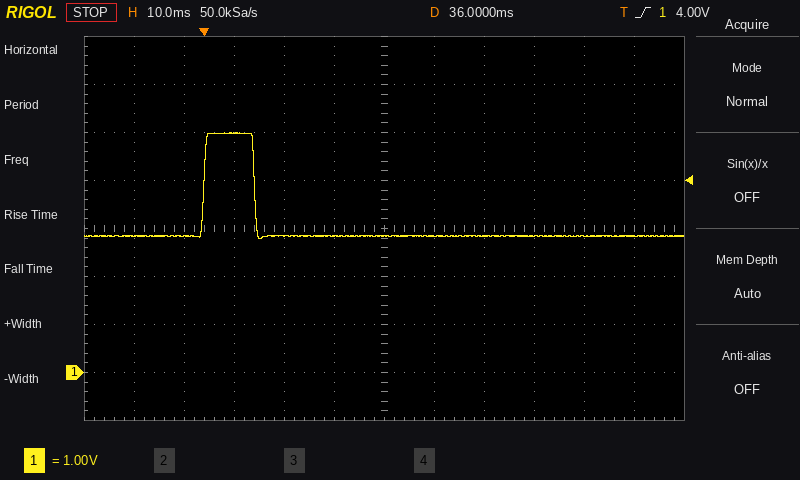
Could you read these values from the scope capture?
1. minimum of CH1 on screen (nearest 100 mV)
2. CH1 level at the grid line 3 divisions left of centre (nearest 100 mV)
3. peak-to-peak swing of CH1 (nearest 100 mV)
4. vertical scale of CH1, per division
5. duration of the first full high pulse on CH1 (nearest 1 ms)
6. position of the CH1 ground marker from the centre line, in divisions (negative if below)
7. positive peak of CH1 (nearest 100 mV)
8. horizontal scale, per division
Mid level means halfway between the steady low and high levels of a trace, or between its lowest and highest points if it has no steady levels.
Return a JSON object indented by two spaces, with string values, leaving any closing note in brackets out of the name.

{
  "minimum of CH1 on screen": "2.8 V",
  "CH1 level at the grid line 3 divisions left of centre": "5.0 V",
  "peak-to-peak swing of CH1": "2.2 V",
  "vertical scale of CH1, per division": "1 V",
  "duration of the first full high pulse on CH1": "10 ms",
  "position of the CH1 ground marker from the centre line, in divisions": "-3.0 div",
  "positive peak of CH1": "5.0 V",
  "horizontal scale, per division": "10 ms"
}
